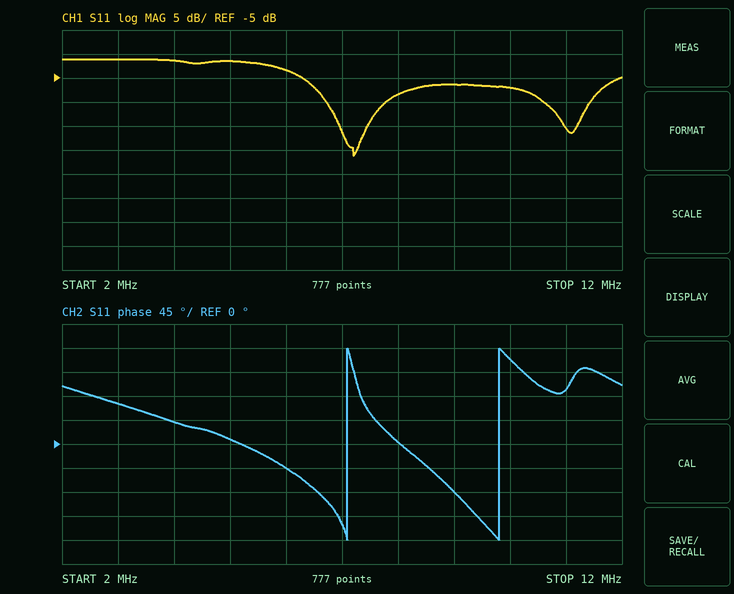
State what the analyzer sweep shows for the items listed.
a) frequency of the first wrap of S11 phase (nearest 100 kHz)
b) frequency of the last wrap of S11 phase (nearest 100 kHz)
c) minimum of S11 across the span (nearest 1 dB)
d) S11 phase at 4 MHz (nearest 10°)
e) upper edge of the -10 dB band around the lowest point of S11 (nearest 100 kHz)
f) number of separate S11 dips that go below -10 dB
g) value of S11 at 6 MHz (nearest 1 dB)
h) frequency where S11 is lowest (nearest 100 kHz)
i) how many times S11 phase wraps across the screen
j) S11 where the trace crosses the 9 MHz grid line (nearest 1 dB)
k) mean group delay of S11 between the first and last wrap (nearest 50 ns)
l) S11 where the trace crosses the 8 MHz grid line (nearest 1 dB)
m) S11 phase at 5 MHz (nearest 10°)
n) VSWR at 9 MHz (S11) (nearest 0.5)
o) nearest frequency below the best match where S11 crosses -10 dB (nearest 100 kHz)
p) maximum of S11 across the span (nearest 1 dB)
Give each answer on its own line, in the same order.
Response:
7.1 MHz
9.8 MHz
-21 dB
40°
7.8 MHz
2
-3 dB
7.2 MHz
2
-6 dB
350 ns
-8 dB
10°
3.0
6.7 MHz
-1 dB
